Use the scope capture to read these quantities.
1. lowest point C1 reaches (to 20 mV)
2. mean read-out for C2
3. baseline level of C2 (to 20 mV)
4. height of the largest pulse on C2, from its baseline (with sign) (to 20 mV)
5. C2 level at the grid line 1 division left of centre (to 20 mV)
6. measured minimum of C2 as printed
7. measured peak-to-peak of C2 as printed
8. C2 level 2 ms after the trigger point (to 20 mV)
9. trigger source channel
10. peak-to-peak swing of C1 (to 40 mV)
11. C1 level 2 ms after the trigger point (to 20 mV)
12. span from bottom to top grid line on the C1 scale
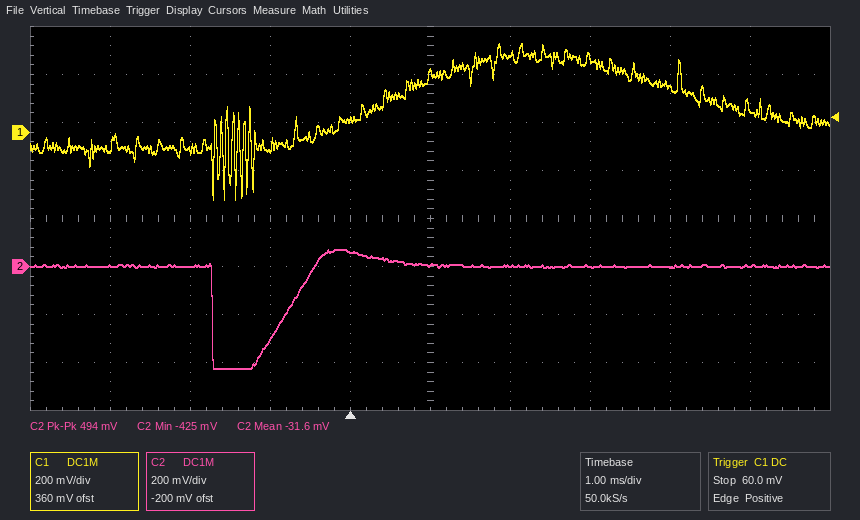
-280 mV
-31.6 mV
0 mV
-420 mV
60 mV
-425 mV
494 mV
0 mV
C1
640 mV
320 mV
1.6 V
